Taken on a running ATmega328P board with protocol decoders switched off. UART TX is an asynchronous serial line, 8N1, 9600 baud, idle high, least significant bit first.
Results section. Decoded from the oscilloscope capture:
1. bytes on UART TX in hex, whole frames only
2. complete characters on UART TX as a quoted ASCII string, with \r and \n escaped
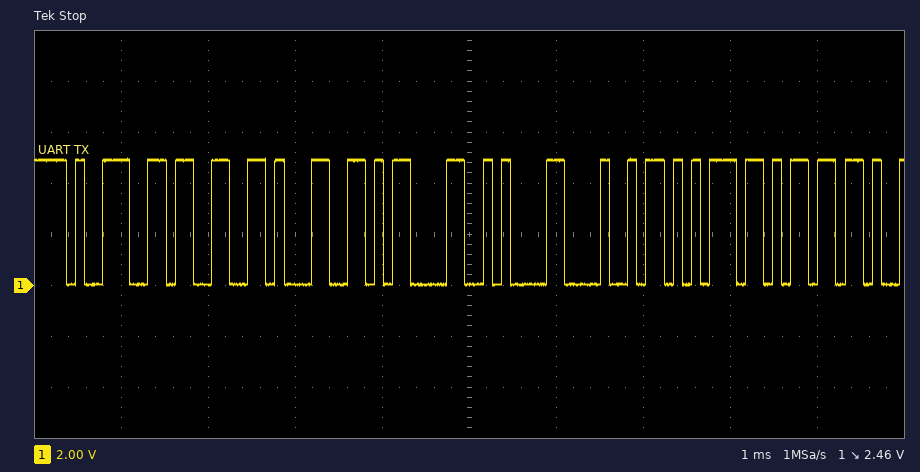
0x39 0x33 0x31 0x0D 0x0A 0x48 0x75 0x6D
"931\r\nHum"
